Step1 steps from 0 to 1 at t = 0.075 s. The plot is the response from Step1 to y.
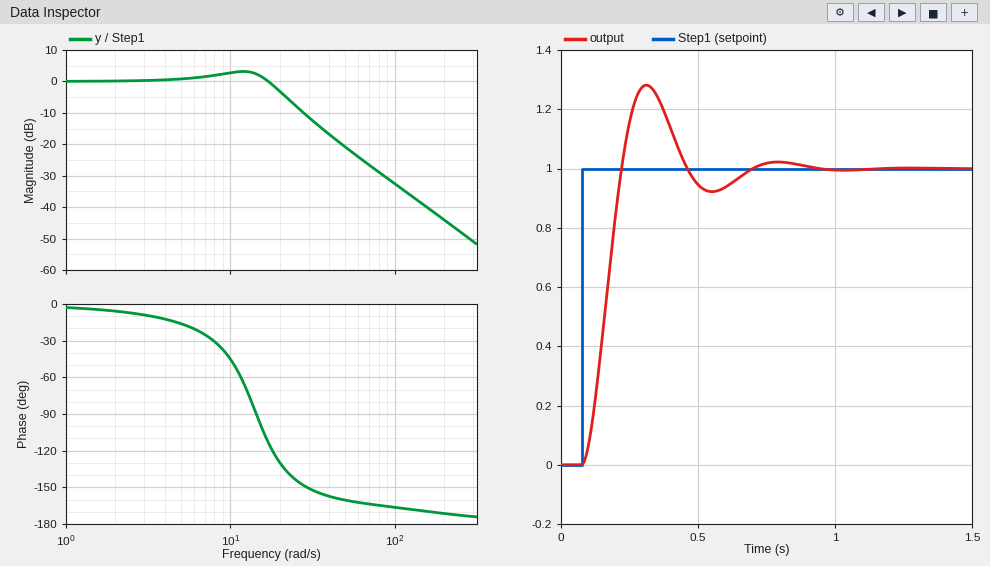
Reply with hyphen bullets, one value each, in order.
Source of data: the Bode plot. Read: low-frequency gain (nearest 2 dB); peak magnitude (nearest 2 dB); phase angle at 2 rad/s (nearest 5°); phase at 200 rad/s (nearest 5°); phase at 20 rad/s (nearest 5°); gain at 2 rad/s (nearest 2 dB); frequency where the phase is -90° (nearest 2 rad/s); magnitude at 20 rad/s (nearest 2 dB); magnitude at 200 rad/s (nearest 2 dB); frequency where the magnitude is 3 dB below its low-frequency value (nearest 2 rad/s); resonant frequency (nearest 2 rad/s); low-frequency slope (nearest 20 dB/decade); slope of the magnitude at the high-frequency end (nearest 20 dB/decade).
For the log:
- 0 dB
- 4 dB
- -5°
- -170°
- -130°
- 0 dB
- 14 rad/s
- -4 dB
- -44 dB
- 20 rad/s
- 12 rad/s
- 0 dB/decade
- -40 dB/decade
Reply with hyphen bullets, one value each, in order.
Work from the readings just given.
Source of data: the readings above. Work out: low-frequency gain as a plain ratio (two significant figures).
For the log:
- 1.0
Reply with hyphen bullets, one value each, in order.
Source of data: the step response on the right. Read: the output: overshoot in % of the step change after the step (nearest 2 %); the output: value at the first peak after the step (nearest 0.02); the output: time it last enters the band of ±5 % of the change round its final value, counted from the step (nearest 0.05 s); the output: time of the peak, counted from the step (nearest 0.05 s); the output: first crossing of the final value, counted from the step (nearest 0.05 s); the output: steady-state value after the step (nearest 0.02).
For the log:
- 28 %
- 1.28
- 0.55 s
- 0.25 s
- 0.15 s
- 1.00
